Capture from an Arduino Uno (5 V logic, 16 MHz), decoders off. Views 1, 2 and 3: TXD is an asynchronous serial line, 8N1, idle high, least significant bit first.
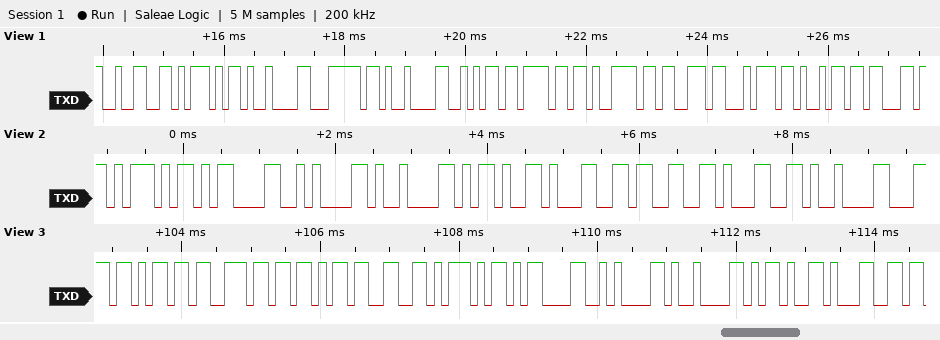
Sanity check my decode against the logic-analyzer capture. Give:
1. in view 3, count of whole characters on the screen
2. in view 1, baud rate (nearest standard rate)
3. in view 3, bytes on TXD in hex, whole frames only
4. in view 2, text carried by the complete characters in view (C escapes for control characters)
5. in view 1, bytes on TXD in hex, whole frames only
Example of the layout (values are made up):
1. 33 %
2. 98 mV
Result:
1. 10
2. 9600 baud
3. 6B 73 5B 33 5D 0D 0A 09 2D 31
4. "]\r\n\t-131\t"
5. 32 5D 09 7C 09 6A 6F 79 73 74 69 63
